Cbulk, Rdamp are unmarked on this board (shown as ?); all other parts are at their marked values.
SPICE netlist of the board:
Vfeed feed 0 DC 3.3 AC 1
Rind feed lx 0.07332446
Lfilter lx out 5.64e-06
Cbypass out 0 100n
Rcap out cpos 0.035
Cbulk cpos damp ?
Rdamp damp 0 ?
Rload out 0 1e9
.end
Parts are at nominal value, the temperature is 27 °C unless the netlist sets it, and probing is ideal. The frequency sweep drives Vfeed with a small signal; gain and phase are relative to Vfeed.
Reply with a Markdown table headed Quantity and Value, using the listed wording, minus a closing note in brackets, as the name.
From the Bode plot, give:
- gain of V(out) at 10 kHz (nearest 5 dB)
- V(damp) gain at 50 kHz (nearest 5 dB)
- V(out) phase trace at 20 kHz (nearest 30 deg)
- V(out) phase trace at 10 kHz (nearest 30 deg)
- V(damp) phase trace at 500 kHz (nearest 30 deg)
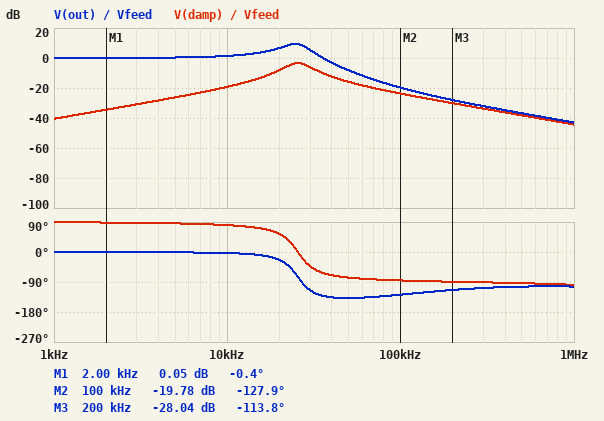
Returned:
| Quantity | Value |
|---|---|
| gain of V(out) at 10 kHz | 0 dB |
| V(damp) gain at 50 kHz | -15 dB |
| V(out) phase trace at 20 kHz | -30 deg |
| V(out) phase trace at 10 kHz | 0 deg |
| V(damp) phase trace at 500 kHz | -90 deg |
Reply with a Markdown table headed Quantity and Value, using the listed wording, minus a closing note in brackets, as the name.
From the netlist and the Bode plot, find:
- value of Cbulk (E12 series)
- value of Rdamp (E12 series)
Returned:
| Quantity | Value |
|---|---|
| value of Cbulk | 6.8 µF |
| value of Rdamp | 0.22 Ω |
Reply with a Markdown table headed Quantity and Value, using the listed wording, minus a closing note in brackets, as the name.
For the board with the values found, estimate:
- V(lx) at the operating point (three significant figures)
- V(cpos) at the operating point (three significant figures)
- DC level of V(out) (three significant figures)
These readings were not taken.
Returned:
| Quantity | Value |
|---|---|
| V(lx) at the operating point | 3.30 V |
| V(cpos) at the operating point | 3.30 V |
| DC level of V(out) | 3.30 V |
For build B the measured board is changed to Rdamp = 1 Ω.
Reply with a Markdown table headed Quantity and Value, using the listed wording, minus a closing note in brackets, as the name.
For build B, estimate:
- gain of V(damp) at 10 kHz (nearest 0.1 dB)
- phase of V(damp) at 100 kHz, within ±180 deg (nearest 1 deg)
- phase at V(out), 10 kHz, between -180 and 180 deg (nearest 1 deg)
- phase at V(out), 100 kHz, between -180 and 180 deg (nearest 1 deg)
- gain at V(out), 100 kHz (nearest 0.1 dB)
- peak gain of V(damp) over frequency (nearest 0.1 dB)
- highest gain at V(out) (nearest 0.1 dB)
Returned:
| Quantity | Value |
|---|---|
| gain of V(damp) at 10 kHz | -7.1 dB |
| phase of V(damp) at 100 kHz, within ±180 deg | -75 deg |
| phase at V(out), 10 kHz, between -180 and 180 deg | -5 deg |
| phase at V(out), 100 kHz, between -180 and 180 deg | -88 deg |
| gain at V(out), 100 kHz | -10.3 dB |
| peak gain of V(damp) over frequency | -0.8 dB |
| highest gain at V(out) | 2.4 dB |
